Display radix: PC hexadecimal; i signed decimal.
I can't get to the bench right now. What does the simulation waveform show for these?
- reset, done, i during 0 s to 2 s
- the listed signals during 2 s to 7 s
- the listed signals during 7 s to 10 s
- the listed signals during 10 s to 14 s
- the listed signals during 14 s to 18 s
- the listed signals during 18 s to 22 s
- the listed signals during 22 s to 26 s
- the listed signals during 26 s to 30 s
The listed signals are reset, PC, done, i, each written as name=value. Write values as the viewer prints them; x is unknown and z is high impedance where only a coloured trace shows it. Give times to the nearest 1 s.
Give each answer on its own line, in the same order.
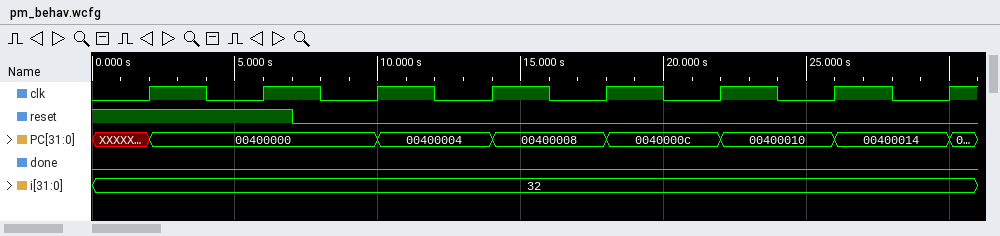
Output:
reset=1, done=0, i=32
reset=1, PC=00400000, done=0, i=32
reset=0, PC=00400000, done=0, i=32
reset=0, PC=00400004, done=0, i=32
reset=0, PC=00400008, done=0, i=32
reset=0, PC=0040000c, done=0, i=32
reset=0, PC=00400010, done=0, i=32
reset=0, PC=00400014, done=0, i=32
